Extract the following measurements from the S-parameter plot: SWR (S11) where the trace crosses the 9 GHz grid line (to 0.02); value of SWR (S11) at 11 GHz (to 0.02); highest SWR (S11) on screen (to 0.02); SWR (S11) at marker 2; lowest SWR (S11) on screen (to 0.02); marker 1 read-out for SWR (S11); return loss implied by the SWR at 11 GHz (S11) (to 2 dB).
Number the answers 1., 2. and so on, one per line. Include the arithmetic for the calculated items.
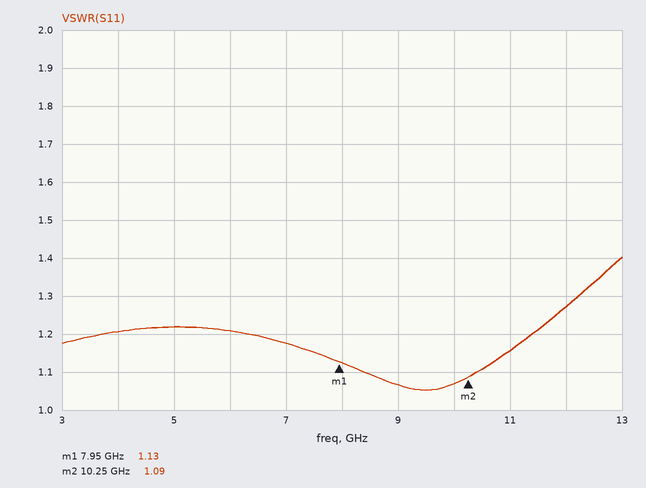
1. 1.06
2. 1.16
3. 1.40
4. 1.09
5. 1.06
6. 1.13
7. −20 log10((1.16 − 1)/(1.16 + 1)) ≈ 22.6 dB, so 22 dB to the nearest 2 dB
